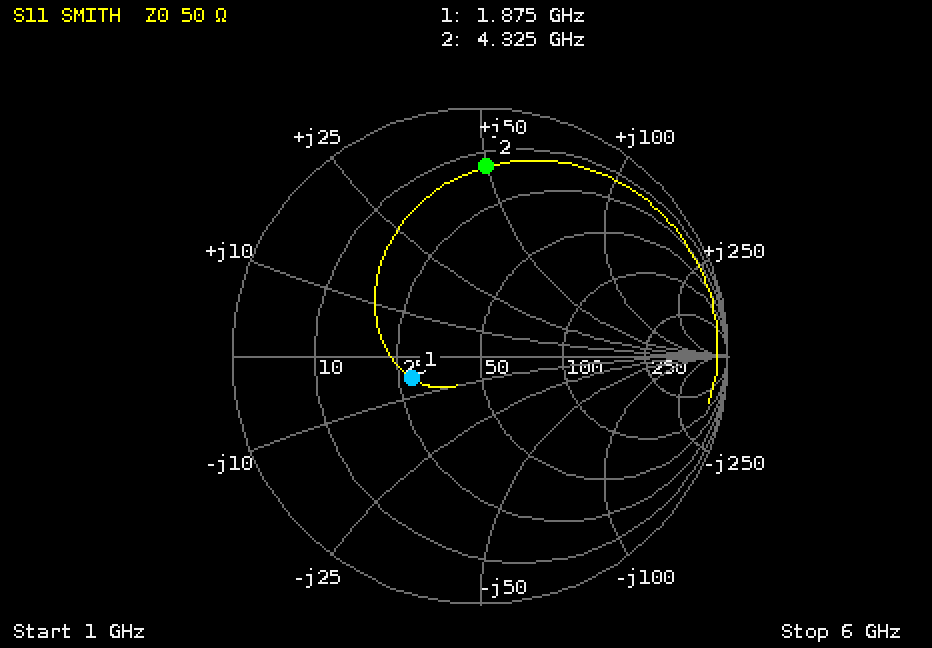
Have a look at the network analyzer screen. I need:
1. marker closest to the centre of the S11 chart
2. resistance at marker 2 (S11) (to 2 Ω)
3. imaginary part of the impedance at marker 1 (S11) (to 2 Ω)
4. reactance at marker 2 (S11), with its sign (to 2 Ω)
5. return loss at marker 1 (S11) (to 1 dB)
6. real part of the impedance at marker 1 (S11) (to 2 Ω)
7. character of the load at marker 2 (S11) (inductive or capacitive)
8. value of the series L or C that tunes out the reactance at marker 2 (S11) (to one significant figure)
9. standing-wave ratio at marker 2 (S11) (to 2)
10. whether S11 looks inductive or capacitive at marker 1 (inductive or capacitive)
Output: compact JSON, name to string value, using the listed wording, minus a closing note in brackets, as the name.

{"marker closest to the centre of the S11 chart": "marker 1", "resistance at marker 2 (S11)": "14 Ω", "imaginary part of the impedance at marker 1 (S11)": "-6 Ω", "reactance at marker 2 (S11), with its sign": "+50 Ω", "return loss at marker 1 (S11)": "11 dB", "real part of the impedance at marker 1 (S11)": "28 Ω", "character of the load at marker 2 (S11)": "inductive", "value of the series L or C that tunes out the reactance at marker 2 (S11)": "700 fF", "standing-wave ratio at marker 2 (S11)": "8", "whether S11 looks inductive or capacitive at marker 1": "capacitive"}
